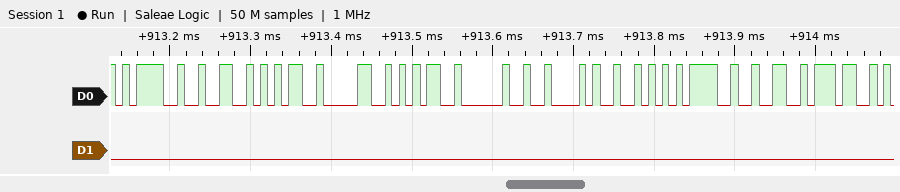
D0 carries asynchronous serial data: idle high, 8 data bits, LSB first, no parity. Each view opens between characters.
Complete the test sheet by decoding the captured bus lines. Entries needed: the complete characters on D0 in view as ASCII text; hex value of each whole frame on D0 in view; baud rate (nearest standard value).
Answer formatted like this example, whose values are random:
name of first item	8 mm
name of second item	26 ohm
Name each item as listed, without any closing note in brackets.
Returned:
the complete characters on D0 in view as ASCII text	"=2505 BR=27"
hex value of each whole frame on D0 in view	3D, 32, 35, 30, 35, 20, 42, 52, 3D, 32, 37
baud rate	115200 baud
